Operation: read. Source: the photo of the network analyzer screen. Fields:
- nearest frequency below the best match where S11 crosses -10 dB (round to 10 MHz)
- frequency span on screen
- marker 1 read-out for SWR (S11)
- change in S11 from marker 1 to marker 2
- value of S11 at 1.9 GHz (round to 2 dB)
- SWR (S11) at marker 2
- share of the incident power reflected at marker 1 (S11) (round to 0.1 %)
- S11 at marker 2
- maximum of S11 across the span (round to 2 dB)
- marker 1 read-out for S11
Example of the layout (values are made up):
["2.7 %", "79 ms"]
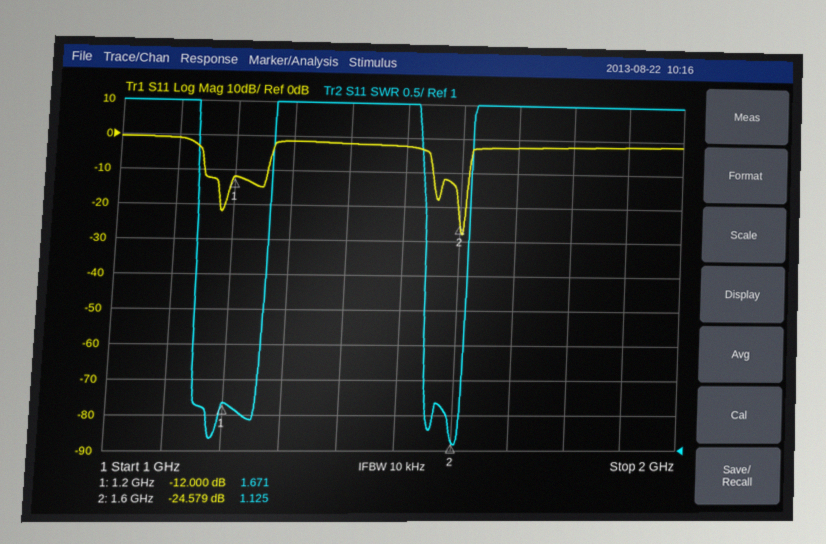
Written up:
["1.55 GHz", "1 GHz", "1.671", "-12.579 dB", "-2 dB", "1.125", "6.3 %", "-24.579 dB", "0 dB", "-12.000 dB"]
